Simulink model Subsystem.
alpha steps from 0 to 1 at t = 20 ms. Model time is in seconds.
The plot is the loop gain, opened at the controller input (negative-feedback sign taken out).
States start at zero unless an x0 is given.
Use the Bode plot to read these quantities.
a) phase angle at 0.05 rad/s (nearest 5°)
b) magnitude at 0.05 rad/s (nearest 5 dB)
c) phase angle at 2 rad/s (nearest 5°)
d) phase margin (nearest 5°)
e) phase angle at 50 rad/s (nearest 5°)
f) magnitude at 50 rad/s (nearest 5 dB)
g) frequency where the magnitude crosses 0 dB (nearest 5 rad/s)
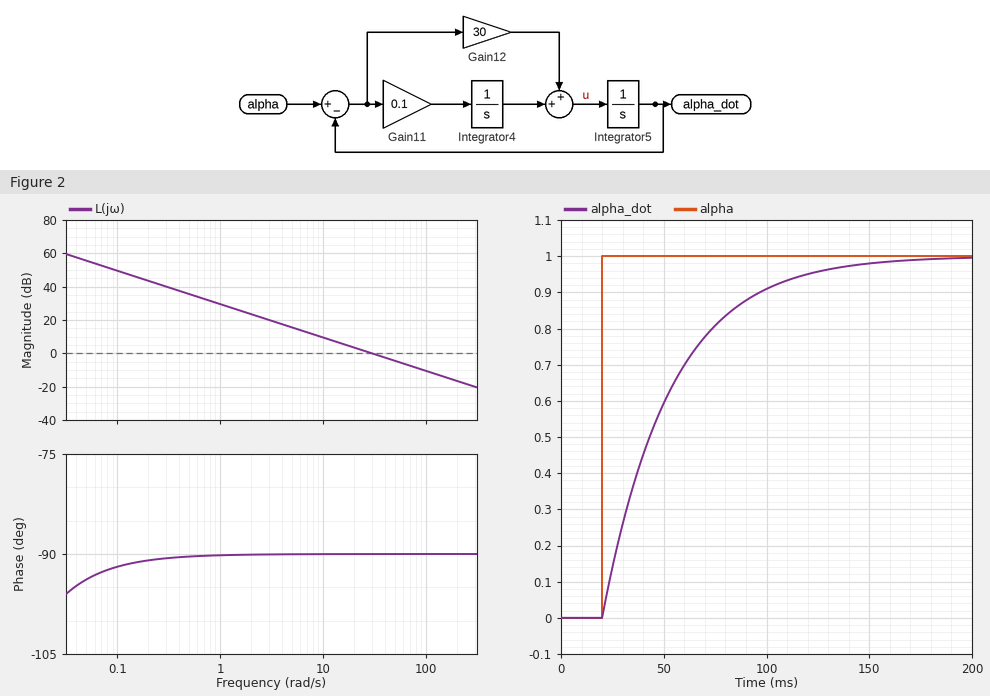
-95°
55 dB
-90°
90°
-90°
-5 dB
30 rad/s
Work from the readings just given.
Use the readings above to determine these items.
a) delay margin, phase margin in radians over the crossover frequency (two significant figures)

0.052 s
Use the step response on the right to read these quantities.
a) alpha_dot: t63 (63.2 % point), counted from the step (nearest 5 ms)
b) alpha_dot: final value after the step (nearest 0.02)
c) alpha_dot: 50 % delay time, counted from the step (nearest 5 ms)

35 ms
1.00
25 ms
